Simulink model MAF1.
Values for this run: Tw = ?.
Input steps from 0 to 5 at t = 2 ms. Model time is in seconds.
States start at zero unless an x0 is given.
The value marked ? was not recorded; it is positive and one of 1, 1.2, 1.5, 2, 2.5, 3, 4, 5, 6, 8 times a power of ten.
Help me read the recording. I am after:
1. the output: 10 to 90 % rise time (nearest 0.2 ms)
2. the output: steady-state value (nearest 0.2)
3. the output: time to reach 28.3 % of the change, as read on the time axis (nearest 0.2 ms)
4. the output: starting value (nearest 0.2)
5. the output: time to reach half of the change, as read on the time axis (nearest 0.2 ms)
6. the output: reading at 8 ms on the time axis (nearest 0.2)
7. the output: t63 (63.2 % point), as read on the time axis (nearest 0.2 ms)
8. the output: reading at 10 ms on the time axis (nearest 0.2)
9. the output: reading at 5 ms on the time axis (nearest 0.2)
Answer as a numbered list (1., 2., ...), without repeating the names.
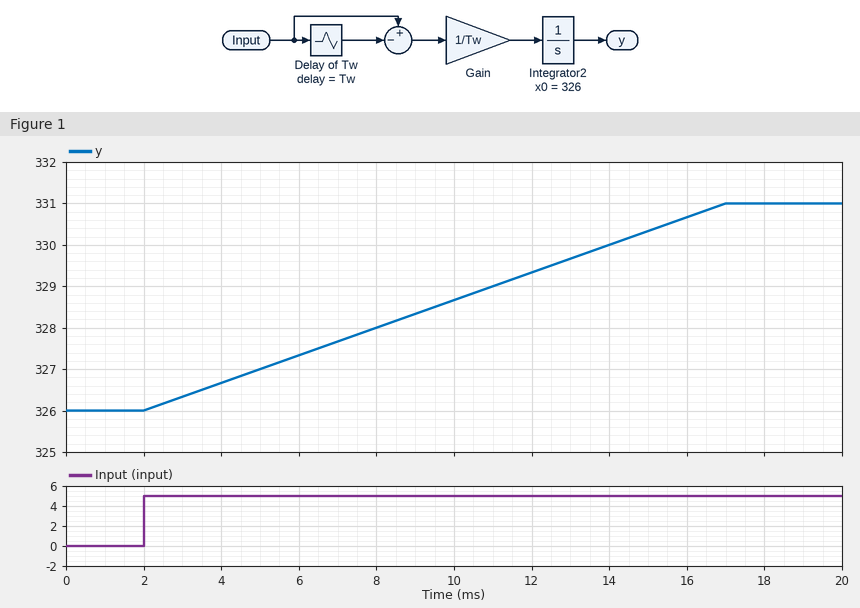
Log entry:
1. 12.0 ms
2. 331.0
3. 6.2 ms
4. 326.0
5. 9.4 ms
6. 328.0
7. 11.4 ms
8. 328.6
9. 327.0
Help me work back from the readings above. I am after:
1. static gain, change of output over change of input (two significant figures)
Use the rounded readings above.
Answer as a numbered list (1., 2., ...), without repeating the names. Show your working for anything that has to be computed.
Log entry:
1. (331 - 326) / (5 - 0) = 1.0
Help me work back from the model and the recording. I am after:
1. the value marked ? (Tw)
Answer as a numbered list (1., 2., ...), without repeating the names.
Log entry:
1. 0.015
